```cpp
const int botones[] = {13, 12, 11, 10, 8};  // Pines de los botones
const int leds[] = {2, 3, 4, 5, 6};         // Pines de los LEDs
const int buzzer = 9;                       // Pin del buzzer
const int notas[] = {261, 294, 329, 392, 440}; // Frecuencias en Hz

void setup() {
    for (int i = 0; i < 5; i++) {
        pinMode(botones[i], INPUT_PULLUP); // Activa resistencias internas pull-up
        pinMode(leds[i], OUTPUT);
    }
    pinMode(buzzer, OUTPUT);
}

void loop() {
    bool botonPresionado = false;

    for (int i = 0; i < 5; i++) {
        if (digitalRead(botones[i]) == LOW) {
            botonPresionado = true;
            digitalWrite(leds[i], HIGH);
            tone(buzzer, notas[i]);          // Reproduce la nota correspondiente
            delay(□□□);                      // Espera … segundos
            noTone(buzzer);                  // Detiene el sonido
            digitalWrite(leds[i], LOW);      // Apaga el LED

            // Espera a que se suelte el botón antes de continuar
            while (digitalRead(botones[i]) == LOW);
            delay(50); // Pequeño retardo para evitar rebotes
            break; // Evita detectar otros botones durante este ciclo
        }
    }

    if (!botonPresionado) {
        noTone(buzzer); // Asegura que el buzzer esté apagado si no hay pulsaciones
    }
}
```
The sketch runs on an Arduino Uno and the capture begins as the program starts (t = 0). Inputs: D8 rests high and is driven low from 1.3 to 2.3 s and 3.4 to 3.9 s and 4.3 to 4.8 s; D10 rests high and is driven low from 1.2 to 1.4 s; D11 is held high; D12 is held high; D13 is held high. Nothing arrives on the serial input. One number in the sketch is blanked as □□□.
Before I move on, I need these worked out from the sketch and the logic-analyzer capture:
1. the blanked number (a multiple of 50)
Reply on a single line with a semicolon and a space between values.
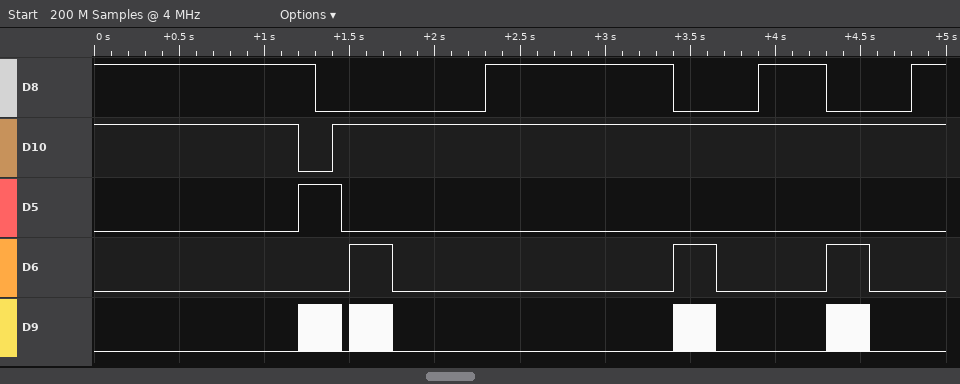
250
